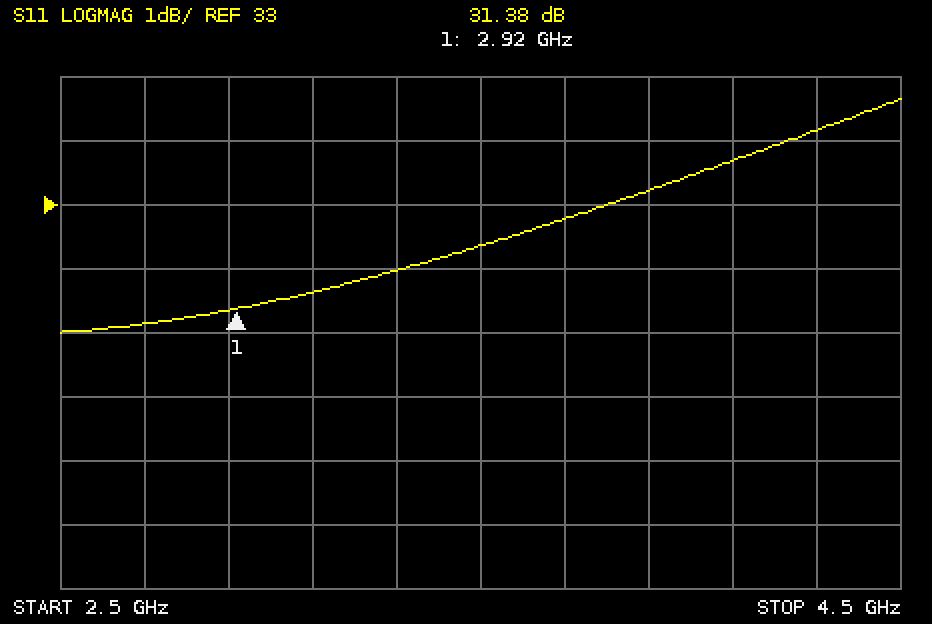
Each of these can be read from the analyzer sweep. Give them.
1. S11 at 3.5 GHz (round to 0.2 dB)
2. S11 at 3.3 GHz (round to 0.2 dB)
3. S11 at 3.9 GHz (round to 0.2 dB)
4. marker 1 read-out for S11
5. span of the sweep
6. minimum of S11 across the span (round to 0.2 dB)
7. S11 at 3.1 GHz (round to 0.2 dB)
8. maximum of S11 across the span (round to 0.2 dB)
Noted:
32.4 dB
32.0 dB
33.2 dB
31.38 dB
2 GHz
31.0 dB
31.6 dB
34.6 dB
